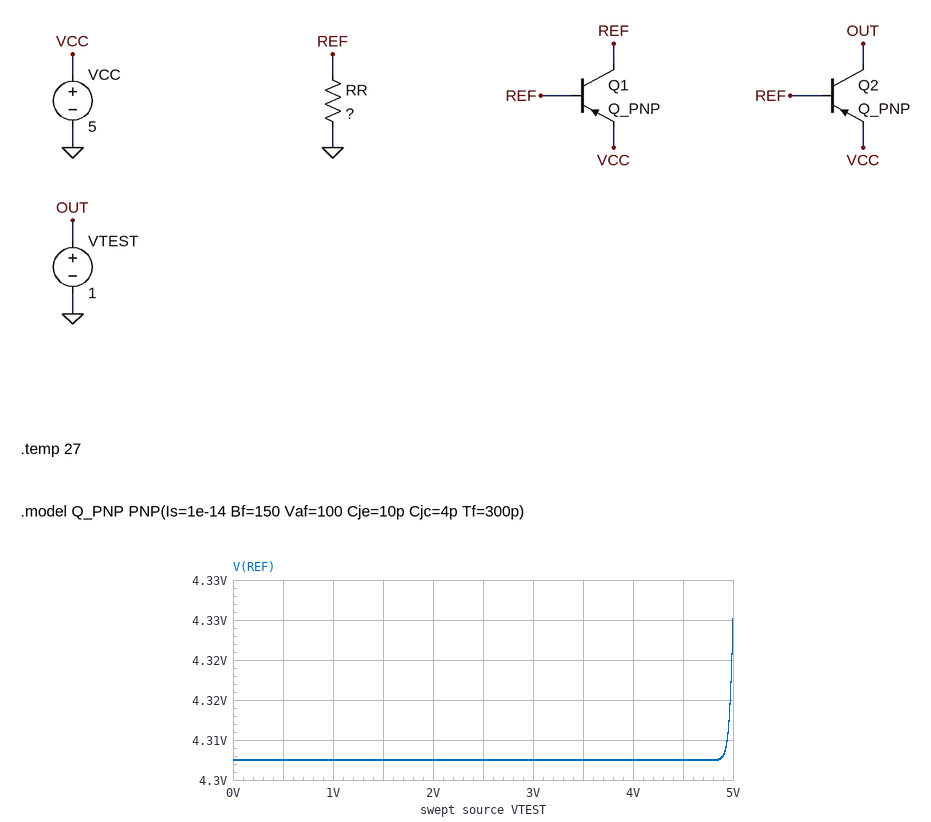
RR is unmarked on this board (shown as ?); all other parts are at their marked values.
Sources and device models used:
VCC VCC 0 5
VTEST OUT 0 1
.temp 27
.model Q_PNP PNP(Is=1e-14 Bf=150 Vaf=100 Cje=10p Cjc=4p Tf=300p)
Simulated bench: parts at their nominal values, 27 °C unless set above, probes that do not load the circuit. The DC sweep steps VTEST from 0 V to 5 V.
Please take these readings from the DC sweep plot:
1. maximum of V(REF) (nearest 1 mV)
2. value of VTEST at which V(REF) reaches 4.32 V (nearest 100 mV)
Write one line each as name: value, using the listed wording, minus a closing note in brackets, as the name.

maximum of V(REF): 4.325 V
value of VTEST at which V(REF) reaches 4.32 V: 5.0 V
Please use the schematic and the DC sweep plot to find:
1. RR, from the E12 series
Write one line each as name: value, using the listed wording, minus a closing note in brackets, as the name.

RR, from the E12 series: 1 kΩ
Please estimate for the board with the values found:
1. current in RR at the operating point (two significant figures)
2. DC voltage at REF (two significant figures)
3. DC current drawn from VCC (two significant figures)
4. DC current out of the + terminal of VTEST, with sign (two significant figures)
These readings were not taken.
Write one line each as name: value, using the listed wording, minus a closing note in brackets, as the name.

current in RR at the operating point: 4.3 mA
DC voltage at REF: 4.3 V
DC current drawn from VCC: 8.7 mA
DC current out of the + terminal of VTEST, with sign: -4.4 mA
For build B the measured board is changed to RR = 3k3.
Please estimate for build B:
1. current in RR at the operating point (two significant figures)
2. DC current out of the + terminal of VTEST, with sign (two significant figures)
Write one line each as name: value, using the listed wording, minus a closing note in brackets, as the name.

current in RR at the operating point: 1.3 mA
DC current out of the + terminal of VTEST, with sign: -1.3 mA
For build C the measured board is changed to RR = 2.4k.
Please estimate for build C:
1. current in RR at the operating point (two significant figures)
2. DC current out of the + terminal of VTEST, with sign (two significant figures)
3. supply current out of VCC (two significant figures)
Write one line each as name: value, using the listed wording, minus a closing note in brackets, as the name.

current in RR at the operating point: 1.8 mA
DC current out of the + terminal of VTEST, with sign: -1.8 mA
supply current out of VCC: 3.6 mA
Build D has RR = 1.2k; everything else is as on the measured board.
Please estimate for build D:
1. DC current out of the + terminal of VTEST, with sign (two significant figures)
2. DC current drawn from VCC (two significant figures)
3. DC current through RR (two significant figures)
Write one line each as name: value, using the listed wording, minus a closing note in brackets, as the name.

DC current out of the + terminal of VTEST, with sign: -3.7 mA
DC current drawn from VCC: 7.3 mA
DC current through RR: 3.6 mA
